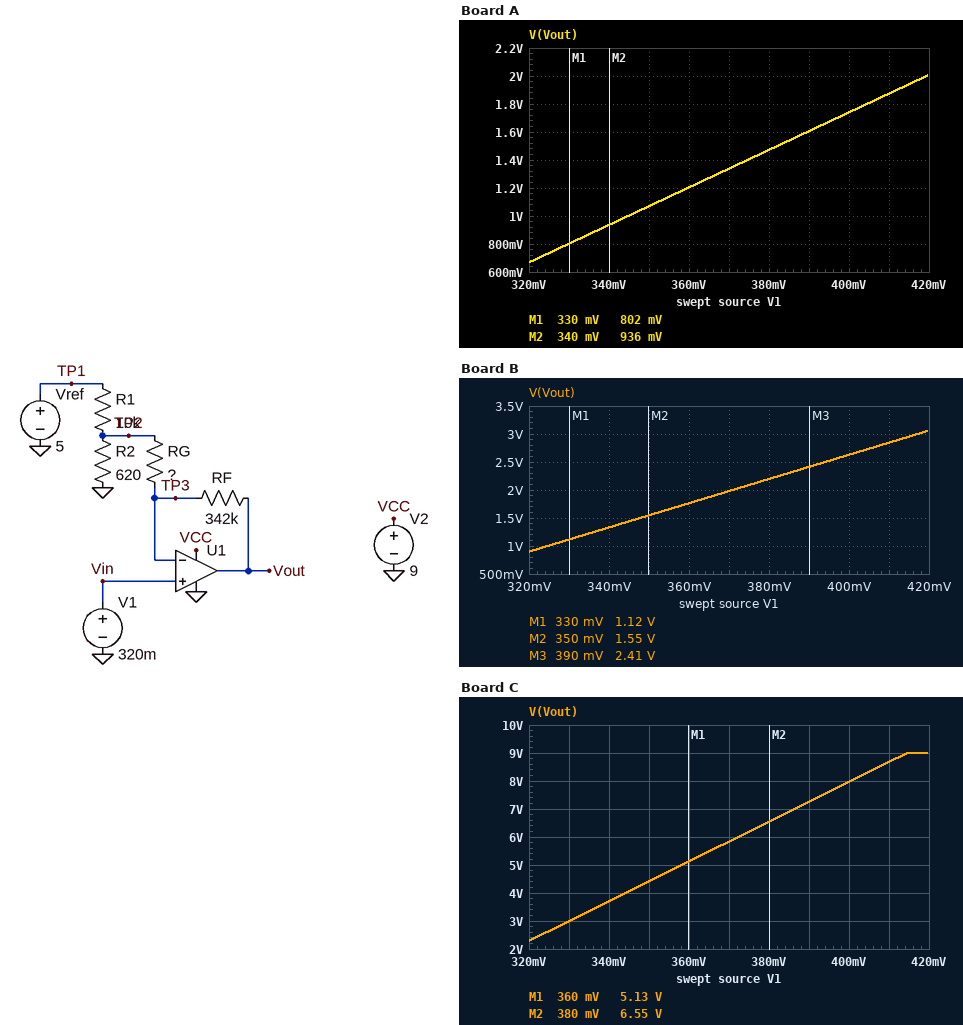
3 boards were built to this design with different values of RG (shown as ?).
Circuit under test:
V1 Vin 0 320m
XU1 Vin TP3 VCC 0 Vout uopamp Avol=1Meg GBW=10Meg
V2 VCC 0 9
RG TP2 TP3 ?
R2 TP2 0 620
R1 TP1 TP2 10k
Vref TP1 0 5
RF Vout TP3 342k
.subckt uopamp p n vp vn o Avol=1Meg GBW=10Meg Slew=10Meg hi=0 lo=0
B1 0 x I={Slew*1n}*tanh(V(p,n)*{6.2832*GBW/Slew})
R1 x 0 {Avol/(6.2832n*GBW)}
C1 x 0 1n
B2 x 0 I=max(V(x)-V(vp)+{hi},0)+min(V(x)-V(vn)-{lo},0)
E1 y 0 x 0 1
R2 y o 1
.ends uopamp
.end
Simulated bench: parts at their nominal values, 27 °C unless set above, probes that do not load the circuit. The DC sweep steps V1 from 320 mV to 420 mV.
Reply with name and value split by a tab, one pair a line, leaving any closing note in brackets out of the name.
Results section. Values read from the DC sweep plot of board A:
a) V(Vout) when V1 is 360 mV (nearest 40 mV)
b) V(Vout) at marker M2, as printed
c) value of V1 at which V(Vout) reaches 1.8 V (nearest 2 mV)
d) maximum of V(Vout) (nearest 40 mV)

V(Vout) when V1 is 360 mV	1.20 V
V(Vout) at marker M2, as printed	936 mV
value of V1 at which V(Vout) reaches 1.8 V	404 mV
maximum of V(Vout)	2.00 V
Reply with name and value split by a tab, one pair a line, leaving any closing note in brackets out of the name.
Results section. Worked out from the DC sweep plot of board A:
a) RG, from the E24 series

RG, from the E24 series	27 kΩ
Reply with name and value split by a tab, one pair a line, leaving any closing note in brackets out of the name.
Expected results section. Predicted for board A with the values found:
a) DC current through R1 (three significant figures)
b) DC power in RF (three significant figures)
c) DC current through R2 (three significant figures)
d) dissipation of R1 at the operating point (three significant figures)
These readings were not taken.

DC current through R1	471 µA
DC power in RF	355 nW
DC current through R2	472 µA
dissipation of R1 at the operating point	2.22 mW
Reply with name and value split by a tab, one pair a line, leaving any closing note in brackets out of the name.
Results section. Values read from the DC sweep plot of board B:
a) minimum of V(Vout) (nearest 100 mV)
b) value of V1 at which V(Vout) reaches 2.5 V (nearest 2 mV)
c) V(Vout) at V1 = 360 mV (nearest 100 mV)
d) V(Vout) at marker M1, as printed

minimum of V(Vout)	900 mV
value of V1 at which V(Vout) reaches 2.5 V	394 mV
V(Vout) at V1 = 360 mV	1.8 V
V(Vout) at marker M1, as printed	1.12 V
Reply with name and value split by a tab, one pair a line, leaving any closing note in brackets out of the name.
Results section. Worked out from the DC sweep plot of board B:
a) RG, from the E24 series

RG, from the E24 series	16 kΩ
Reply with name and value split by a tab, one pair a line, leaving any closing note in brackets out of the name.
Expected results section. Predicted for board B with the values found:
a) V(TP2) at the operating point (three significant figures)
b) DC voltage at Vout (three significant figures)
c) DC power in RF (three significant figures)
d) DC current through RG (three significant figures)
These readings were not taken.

V(TP2) at the operating point	293 mV
DC voltage at Vout	899 mV
DC power in RF	982 nW
DC current through RG	1.69 µA
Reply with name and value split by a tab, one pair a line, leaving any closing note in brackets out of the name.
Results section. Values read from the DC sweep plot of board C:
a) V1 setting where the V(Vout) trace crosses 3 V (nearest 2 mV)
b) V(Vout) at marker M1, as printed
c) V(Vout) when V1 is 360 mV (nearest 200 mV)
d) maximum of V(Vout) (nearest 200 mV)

V1 setting where the V(Vout) trace crosses 3 V	330 mV
V(Vout) at marker M1, as printed	5.13 V
V(Vout) when V1 is 360 mV	5.2 V
maximum of V(Vout)	9.0 V
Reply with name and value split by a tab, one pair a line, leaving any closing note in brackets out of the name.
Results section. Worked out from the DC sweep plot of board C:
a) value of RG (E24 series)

value of RG	4.3 kΩ
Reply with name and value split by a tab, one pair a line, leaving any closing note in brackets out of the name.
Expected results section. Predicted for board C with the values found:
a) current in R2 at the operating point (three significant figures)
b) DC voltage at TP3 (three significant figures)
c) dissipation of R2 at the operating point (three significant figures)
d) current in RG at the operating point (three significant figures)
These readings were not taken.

current in R2 at the operating point	476 µA
DC voltage at TP3	320 mV
dissipation of R2 at the operating point	141 µW
current in RG at the operating point	5.75 µA
